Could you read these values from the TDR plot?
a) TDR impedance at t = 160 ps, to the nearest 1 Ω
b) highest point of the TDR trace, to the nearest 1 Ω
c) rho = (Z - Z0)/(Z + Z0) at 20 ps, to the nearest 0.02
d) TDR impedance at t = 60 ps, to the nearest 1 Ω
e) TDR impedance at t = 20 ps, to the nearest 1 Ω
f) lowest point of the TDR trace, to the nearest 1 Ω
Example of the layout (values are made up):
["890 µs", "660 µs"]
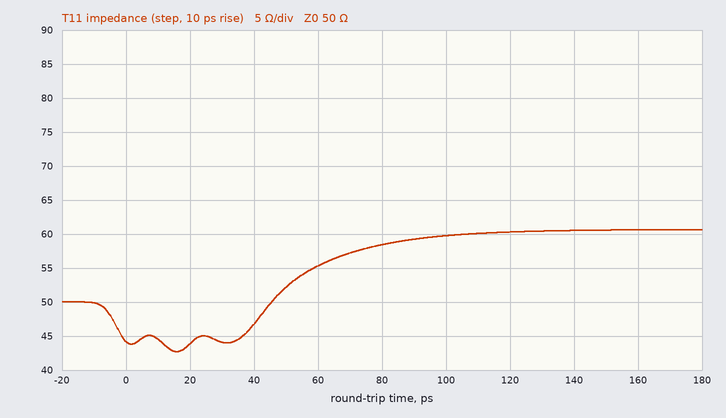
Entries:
["61 Ω", "61 Ω", "-0.06", "55 Ω", "44 Ω", "43 Ω"]
